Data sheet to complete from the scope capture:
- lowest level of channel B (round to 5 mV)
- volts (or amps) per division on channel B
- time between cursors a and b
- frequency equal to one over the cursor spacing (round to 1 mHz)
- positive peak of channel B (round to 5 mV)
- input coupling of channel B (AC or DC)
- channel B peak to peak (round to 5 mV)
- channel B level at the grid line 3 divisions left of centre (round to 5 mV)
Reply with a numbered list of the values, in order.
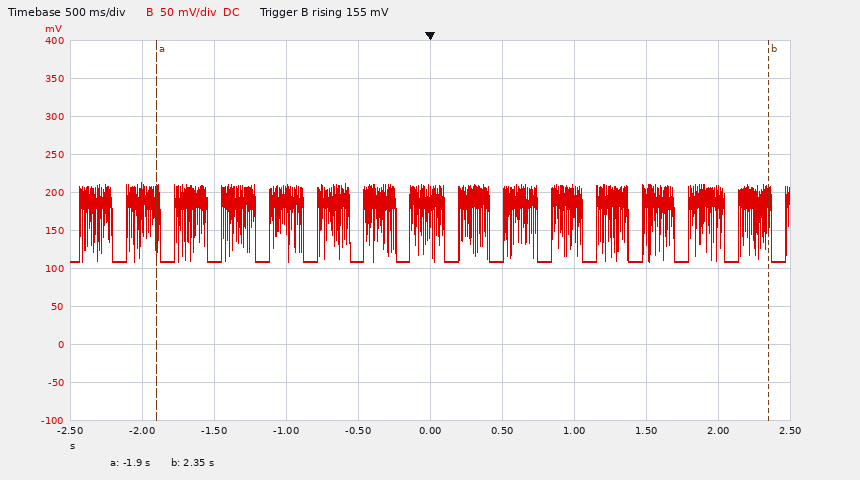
1. 110 mV
2. 50 mV
3. 4.25 s
4. 235 mHz
5. 215 mV
6. DC
7. 105 mV
8. 110 mV
